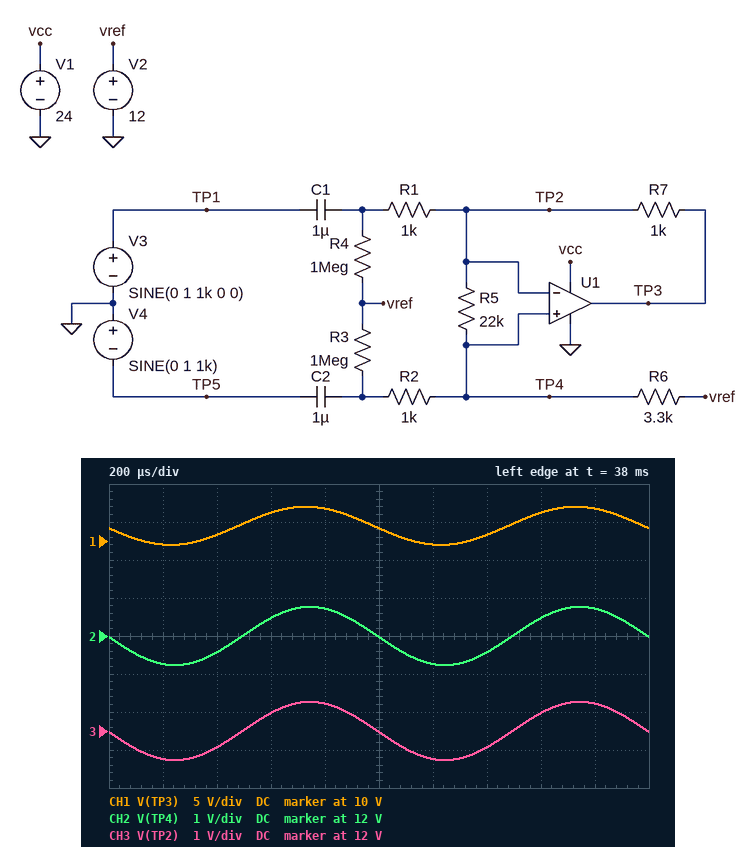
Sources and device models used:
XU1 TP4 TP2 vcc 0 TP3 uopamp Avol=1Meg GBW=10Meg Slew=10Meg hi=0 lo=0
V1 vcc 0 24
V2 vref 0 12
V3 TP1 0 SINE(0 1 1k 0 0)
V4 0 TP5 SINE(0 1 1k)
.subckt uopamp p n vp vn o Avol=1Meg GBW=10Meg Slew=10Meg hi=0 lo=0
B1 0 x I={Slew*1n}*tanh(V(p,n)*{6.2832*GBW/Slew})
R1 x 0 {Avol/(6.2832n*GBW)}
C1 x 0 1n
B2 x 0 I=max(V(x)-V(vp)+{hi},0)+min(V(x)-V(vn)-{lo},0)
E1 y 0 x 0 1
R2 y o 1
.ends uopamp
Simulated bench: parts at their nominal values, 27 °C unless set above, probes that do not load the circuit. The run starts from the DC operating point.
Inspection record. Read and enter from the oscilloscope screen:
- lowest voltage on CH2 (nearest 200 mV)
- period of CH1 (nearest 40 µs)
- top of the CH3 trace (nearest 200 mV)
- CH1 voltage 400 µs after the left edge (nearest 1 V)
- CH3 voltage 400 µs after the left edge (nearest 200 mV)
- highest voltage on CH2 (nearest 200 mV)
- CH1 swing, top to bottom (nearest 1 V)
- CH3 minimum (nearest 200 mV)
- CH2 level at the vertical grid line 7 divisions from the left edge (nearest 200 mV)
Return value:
11.2 V
1.00 ms
12.8 V
11 V
11.6 V
12.8 V
5 V
11.2 V
11.6 V
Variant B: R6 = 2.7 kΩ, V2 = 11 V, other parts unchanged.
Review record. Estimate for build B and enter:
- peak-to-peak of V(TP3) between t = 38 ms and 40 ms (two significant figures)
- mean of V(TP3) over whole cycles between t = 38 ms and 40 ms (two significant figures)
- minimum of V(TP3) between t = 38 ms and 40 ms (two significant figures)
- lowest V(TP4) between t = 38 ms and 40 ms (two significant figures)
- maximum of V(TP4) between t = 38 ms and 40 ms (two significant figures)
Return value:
4.9 V
11 V
8.6 V
10 V
12 V
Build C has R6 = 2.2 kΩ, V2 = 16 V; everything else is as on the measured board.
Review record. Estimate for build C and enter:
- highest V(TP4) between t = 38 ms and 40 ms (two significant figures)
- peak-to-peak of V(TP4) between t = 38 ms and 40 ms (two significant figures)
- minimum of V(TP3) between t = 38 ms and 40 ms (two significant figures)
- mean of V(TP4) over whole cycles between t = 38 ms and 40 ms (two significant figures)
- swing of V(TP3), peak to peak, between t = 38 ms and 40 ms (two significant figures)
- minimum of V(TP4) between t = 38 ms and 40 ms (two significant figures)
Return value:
17 V
1.4 V
14 V
16 V
4.7 V
15 V
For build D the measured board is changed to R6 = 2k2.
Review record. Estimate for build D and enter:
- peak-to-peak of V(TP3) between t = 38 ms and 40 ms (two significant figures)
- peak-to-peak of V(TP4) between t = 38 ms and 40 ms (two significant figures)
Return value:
4.7 V
1.4 V
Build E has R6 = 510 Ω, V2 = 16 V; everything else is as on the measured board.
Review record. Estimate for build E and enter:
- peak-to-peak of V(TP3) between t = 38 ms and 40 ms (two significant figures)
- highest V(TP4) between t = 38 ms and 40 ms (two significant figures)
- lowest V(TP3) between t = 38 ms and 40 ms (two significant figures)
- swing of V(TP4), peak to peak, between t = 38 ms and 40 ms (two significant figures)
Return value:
3.3 V
16 V
14 V
670 mV
